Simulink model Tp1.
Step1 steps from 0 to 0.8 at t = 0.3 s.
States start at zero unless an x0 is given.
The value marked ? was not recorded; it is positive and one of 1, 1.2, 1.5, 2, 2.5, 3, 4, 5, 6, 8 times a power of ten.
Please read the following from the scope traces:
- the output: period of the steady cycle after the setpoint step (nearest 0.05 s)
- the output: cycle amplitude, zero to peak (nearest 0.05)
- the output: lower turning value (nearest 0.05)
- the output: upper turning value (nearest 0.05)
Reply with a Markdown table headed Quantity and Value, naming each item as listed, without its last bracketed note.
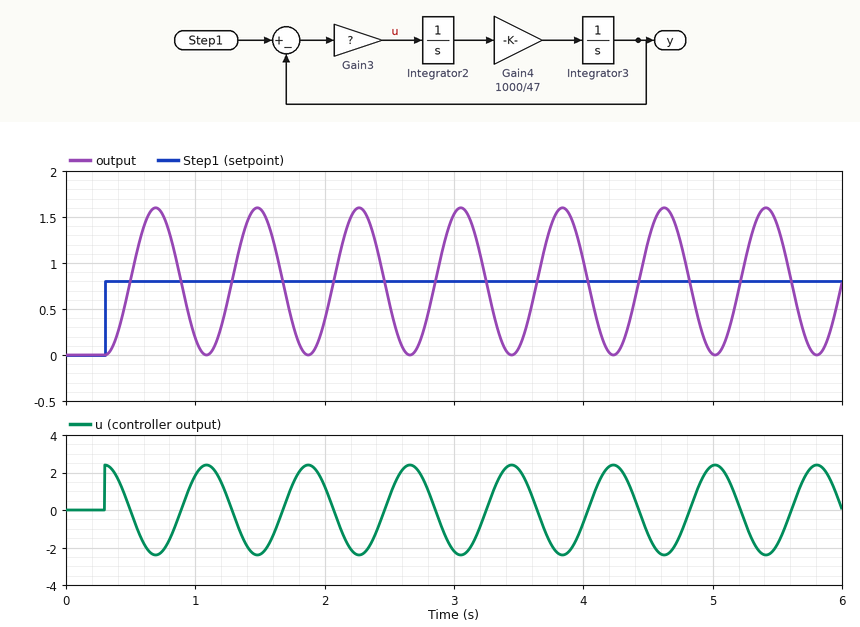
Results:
| Quantity | Value |
|---|---|
| the output: period of the steady cycle after the setpoint step | 0.80 s |
| the output: cycle amplitude, zero to peak | 0.80 |
| the output: lower turning value | 0.00 |
| the output: upper turning value | 1.60 |
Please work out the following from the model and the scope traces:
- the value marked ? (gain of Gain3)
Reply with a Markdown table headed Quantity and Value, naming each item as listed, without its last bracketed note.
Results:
| Quantity | Value |
|---|---|
| the value marked ? | 3 |
